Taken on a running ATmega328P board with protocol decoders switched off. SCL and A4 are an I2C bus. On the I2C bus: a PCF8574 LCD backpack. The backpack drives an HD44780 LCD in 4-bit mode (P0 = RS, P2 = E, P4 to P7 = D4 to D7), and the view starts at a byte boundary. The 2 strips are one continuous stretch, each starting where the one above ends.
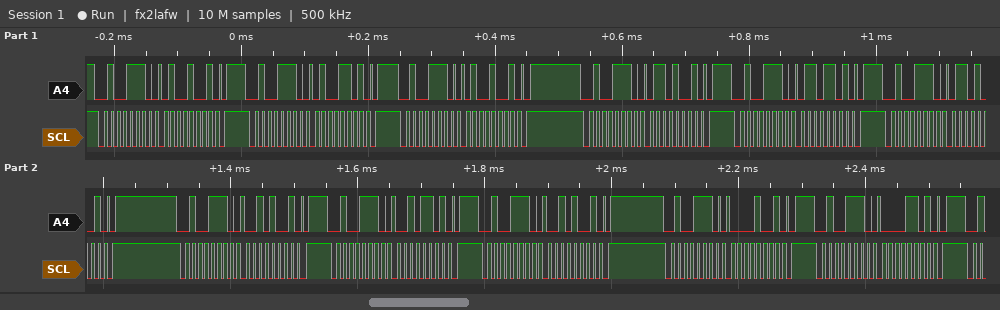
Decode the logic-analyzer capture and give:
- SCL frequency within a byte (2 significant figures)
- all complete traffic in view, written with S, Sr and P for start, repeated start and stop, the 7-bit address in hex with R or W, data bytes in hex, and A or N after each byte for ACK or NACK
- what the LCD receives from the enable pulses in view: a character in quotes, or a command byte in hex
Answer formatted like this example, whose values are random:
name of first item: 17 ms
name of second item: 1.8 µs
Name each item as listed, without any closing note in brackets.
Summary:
SCL frequency within a byte: 100 kHz
all complete traffic in view, written with S, Sr and P for start, repeated start and stop, the 7-bit address in hex with R or W, data bytes in hex, and A or N after each byte for ACK or NACK: S 27W A 49 A P S 27W A 4D A P S 27W A 49 A P S 27W A 69 A P S 27W A 6D A P S 27W A 69 A P S 27W A 29 A P S 27W A 2D A P S 27W A 29 A P S 27W A 09 A P S 27W A 0D A P
what the LCD receives from the enable pulses in view: a character in quotes, or a command byte in hex: 'F'
